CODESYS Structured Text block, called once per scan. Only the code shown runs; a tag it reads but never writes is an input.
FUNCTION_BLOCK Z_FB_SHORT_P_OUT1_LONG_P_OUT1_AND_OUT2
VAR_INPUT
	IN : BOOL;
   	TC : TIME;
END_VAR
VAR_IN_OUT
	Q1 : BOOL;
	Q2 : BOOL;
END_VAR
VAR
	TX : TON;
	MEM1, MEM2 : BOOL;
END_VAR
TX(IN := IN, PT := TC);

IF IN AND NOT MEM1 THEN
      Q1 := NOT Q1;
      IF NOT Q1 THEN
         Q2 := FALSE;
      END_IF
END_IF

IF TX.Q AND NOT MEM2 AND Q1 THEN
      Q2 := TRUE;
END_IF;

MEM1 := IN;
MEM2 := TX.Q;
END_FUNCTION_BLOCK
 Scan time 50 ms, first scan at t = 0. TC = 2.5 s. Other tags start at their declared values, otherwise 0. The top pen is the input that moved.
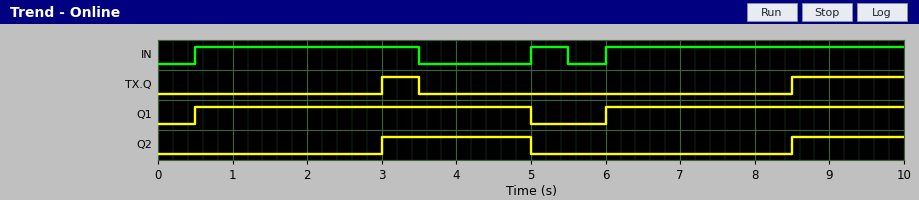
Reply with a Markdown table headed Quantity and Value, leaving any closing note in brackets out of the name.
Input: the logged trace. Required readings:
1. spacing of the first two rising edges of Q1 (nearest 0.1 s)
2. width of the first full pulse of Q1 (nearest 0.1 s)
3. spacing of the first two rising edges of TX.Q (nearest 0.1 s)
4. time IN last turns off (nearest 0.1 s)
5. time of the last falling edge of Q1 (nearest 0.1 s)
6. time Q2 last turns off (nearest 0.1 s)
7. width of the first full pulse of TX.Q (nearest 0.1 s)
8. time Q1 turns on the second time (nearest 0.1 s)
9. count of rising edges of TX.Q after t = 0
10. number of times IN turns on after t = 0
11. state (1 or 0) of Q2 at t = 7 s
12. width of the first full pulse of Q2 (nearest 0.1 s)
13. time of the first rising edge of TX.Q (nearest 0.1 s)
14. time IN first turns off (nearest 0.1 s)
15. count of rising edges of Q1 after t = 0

| Quantity | Value |
|---|---|
| spacing of the first two rising edges of Q1 | 5.5 s |
| width of the first full pulse of Q1 | 4.5 s |
| spacing of the first two rising edges of TX.Q | 5.5 s |
| time IN last turns off | 5.5 s |
| time of the last falling edge of Q1 | 5.0 s |
| time Q2 last turns off | 5.0 s |
| width of the first full pulse of TX.Q | 0.5 s |
| time Q1 turns on the second time | 6.0 s |
| count of rising edges of TX.Q after t = 0 | 2 |
| number of times IN turns on after t = 0 | 3 |
| state (1 or 0) of Q2 at t = 7 s | 0 |
| width of the first full pulse of Q2 | 2.0 s |
| time of the first rising edge of TX.Q | 3.0 s |
| time IN first turns off | 3.5 s |
| count of rising edges of Q1 after t = 0 | 2 |
